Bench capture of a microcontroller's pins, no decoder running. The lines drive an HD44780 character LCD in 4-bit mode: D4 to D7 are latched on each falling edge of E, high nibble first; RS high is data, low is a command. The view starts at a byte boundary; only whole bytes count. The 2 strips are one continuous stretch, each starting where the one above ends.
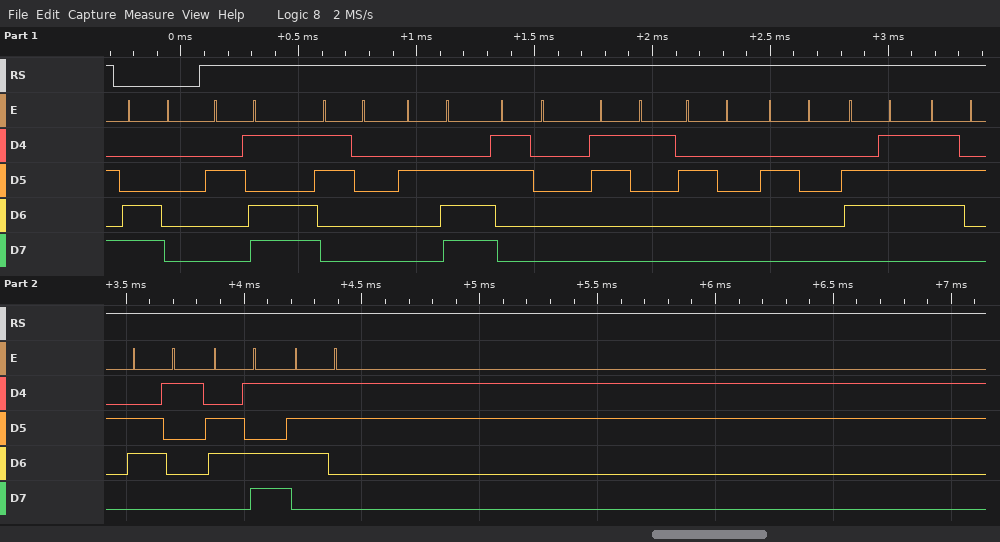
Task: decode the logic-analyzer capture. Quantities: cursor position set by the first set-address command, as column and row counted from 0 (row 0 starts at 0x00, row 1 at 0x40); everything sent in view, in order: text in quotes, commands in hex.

column 0, row 1
0xC0 "-0.01  grams"
